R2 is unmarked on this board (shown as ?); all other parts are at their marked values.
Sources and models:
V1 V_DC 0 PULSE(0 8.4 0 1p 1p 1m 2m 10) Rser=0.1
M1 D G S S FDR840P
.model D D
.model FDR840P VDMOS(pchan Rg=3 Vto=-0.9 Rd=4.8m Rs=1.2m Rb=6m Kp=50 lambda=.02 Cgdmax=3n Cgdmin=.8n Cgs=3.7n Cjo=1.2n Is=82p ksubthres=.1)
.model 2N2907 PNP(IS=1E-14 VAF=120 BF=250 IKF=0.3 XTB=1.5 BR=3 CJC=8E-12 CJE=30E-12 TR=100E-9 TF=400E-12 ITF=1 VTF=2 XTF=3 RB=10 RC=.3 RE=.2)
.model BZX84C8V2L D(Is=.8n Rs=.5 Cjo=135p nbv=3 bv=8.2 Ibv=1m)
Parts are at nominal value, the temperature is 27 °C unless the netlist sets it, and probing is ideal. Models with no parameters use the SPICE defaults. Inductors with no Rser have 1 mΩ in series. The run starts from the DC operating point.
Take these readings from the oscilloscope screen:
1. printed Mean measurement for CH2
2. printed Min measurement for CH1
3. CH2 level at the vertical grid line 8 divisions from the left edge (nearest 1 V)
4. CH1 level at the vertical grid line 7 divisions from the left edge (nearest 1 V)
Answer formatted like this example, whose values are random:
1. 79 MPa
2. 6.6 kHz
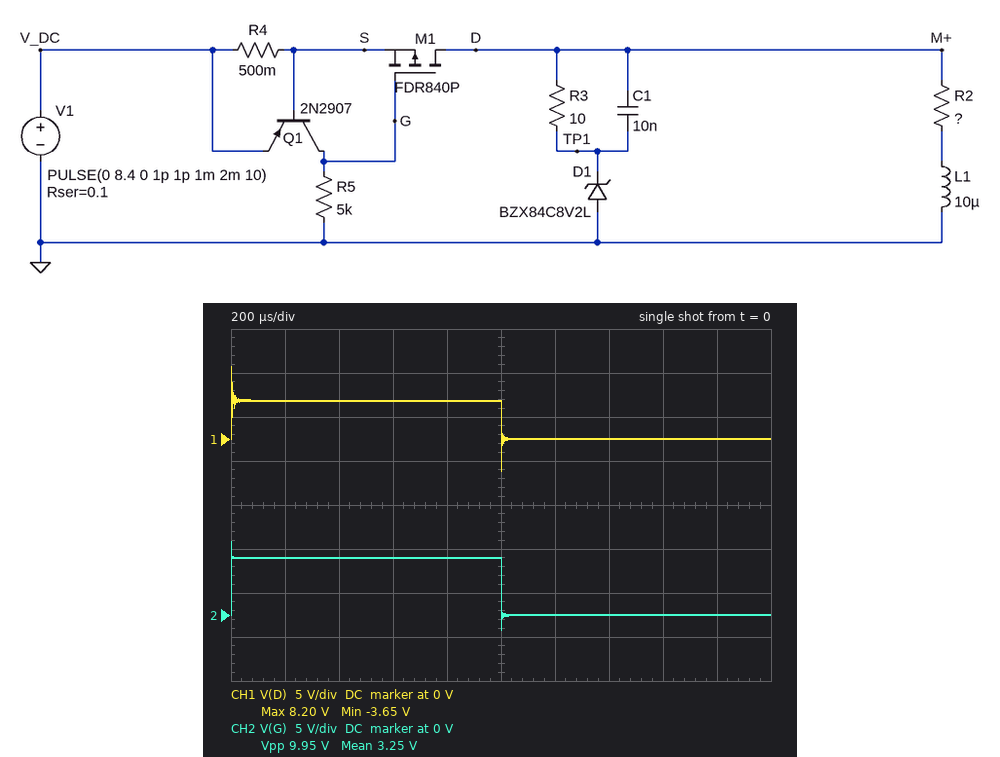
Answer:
1. 3.25 V
2. -3.65 V
3. 0 V
4. 0 V
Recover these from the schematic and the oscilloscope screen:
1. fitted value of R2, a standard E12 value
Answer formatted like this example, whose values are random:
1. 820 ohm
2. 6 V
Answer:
1. 3.3 Ω
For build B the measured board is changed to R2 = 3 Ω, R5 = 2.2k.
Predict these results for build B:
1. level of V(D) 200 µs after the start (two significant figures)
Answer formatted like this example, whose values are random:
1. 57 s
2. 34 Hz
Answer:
1. 4.1 V
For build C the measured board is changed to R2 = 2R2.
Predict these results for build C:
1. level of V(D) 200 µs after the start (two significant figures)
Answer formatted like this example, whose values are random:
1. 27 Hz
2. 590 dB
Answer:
1. 2.9 V
